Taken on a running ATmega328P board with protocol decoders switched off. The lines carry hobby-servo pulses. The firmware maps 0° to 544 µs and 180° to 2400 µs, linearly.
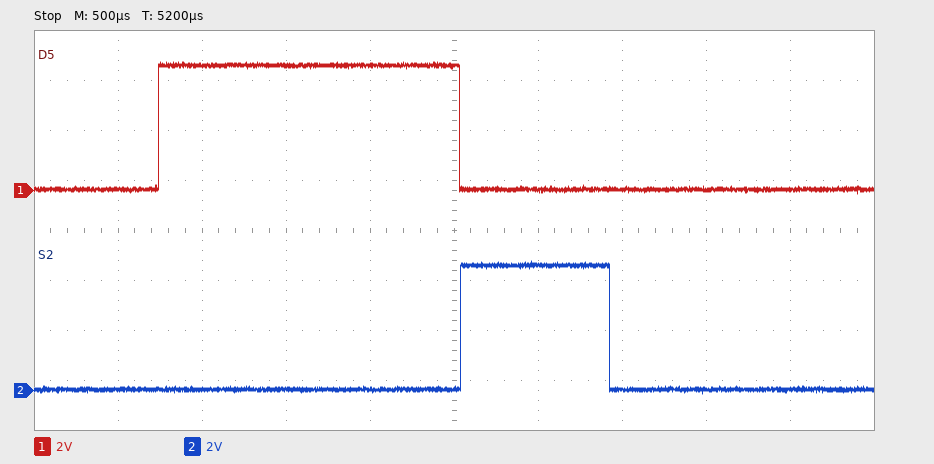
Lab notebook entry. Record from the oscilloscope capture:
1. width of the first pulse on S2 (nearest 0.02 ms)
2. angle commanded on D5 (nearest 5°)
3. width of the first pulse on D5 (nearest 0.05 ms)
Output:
0.88 ms
120°
1.80 ms
